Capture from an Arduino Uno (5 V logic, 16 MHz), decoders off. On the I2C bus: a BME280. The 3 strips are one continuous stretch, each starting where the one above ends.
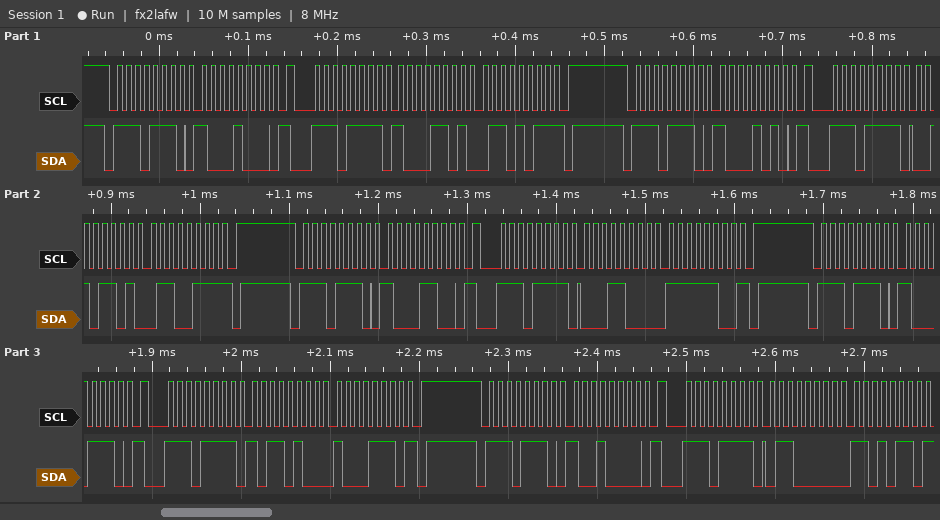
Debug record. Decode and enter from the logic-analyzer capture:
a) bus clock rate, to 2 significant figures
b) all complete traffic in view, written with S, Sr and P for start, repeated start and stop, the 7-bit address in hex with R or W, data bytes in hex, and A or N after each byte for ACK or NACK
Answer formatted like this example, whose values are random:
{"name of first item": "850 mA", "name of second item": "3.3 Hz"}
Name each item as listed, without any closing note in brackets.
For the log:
{"bus clock rate, to 2 significant figures": "100 kHz", "all complete traffic in view, written with S, Sr and P for start, repeated start and stop, the 7-bit address in hex with R or W, data bytes in hex, and A or N after each byte for ACK or NACK": "S 77W A 88 A Sr 77R A 8D A 6B N P S 77W A 8A A Sr 77R A 2D A 67 N P S 77W A 8C A Sr 77R A 18 A FC N P S 77W A 8E A Sr 77R A B4 A 8E N P S 77W A 90 A Sr 77R A 60 A D6 N"}
